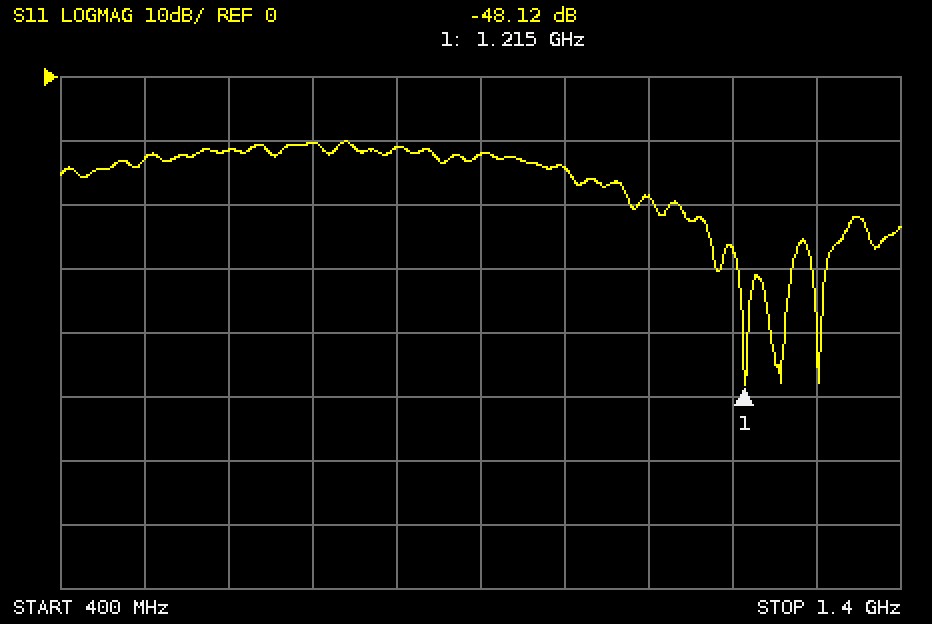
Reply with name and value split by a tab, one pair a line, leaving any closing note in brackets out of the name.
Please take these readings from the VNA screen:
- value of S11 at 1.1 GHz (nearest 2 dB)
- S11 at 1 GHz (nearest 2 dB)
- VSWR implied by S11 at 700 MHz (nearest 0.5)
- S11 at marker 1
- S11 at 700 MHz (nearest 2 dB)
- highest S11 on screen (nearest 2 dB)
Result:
value of S11 at 1.1 GHz	-18 dB
S11 at 1 GHz	-14 dB
VSWR implied by S11 at 700 MHz	2.0
S11 at marker 1	-48.12 dB
S11 at 700 MHz	-10 dB
highest S11 on screen	-10 dB
